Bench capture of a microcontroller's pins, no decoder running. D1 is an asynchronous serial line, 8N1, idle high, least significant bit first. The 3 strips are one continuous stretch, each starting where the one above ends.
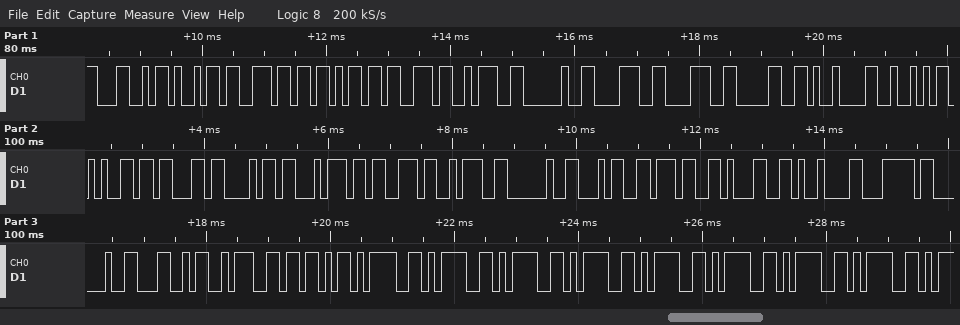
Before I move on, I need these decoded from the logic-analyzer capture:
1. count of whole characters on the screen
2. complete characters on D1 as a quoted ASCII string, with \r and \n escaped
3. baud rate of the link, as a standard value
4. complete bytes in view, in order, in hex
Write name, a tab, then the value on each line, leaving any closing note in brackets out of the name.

count of whole characters on the screen	36
complete characters on D1 as a quoted ASCII string, with \r and \n escaped	"Links: 880\tRechts: 471\t| L:[========"
baud rate of the link, as a standard value	9600 baud
complete bytes in view, in order, in hex	0x4C 0x69 0x6E 0x6B 0x73 0x3A 0x20 0x38 0x38 0x30 0x09 0x52 0x65 0x63 0x68 0x74 0x73 0x3A 0x20 0x34 0x37 0x31 0x09 0x7C 0x20 0x4C 0x3A 0x5B 0x3D 0x3D 0x3D 0x3D 0x3D 0x3D 0x3D 0x3D
